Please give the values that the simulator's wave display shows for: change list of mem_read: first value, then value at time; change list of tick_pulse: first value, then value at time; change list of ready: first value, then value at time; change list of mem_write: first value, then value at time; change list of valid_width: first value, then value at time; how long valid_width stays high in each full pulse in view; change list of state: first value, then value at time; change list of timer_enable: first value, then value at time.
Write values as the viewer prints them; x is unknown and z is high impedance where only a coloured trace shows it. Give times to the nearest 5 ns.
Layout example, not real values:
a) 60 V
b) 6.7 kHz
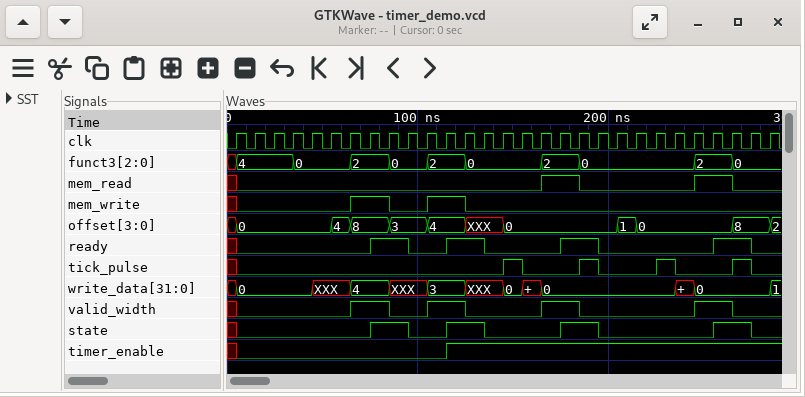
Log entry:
a) x, 0 at 5 ns, 1 at 165 ns, 0 at 185 ns, 1 at 245 ns, 0 at 265 ns
b) x, 0 at 5 ns, 1 at 145 ns, 0 at 155 ns, 1 at 185 ns, 0 at 195 ns, 1 at 225 ns, 0 at 235 ns, 1 at 265 ns, 0 at 275 ns
c) x, 0 at 5 ns, 1 at 75 ns, 0 at 95 ns, 1 at 115 ns, 0 at 135 ns, 1 at 175 ns, 0 at 195 ns, 1 at 255 ns, 0 at 275 ns
d) x, 0 at 5 ns, 1 at 65 ns, 0 at 85 ns, 1 at 105 ns, 0 at 125 ns
e) x, 0 at 5 ns, 1 at 65 ns, 0 at 85 ns, 1 at 105 ns, 0 at 125 ns, 1 at 165 ns, 0 at 185 ns, 1 at 245 ns, 0 at 265 ns
f) 20 ns, 20 ns, 20 ns, 20 ns
g) x, 0 at 5 ns, 1 at 75 ns, 0 at 95 ns, 1 at 115 ns, 0 at 135 ns, 1 at 175 ns, 0 at 195 ns, 1 at 255 ns, 0 at 275 ns
h) x, 0 at 5 ns, 1 at 115 ns
